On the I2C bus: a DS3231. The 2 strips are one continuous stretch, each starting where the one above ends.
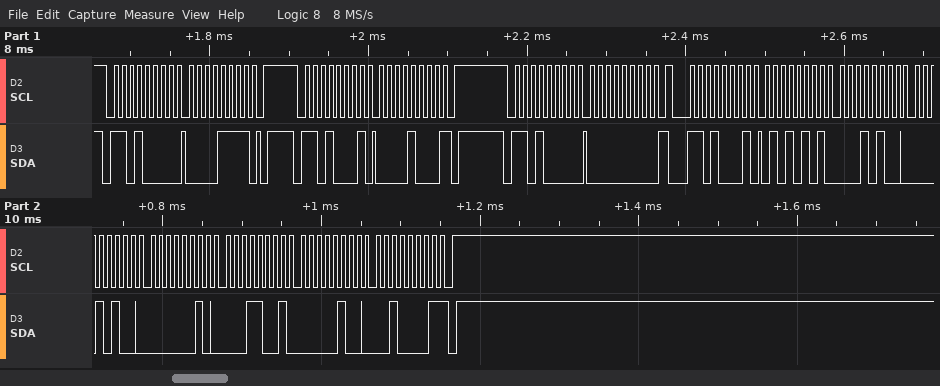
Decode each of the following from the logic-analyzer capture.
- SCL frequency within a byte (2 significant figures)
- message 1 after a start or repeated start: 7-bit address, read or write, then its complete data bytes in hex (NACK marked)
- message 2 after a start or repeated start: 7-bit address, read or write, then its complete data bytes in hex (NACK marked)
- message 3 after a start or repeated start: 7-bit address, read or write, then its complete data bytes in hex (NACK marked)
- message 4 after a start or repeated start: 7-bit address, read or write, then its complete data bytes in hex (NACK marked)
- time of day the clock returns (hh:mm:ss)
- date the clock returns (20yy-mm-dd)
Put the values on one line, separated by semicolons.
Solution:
100 kHz; 0x68 write: 0F; 0x68 read: 08 NACK; 0x68 write: 00; 0x68 read: 55 14 14 02 19 04 21 NACK; 14:14:55; 2021-04-19
